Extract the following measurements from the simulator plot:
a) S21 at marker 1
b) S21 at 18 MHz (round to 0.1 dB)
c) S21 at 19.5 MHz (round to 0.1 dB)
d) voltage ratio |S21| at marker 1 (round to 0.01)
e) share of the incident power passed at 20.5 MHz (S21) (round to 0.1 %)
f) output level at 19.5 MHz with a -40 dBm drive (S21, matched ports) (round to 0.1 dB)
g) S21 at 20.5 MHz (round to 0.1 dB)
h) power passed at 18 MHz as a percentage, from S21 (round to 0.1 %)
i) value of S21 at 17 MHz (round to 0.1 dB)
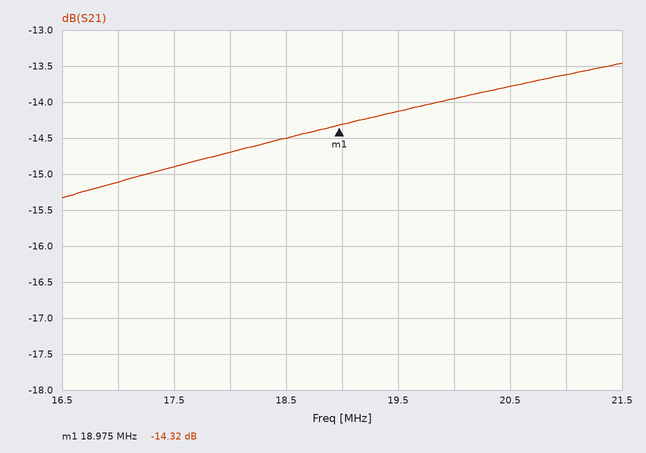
-14.32 dB
-14.7 dB
-14.1 dB
0.19
4.2 %
-54.1 dBm
-13.8 dB
3.4 %
-15.1 dB
